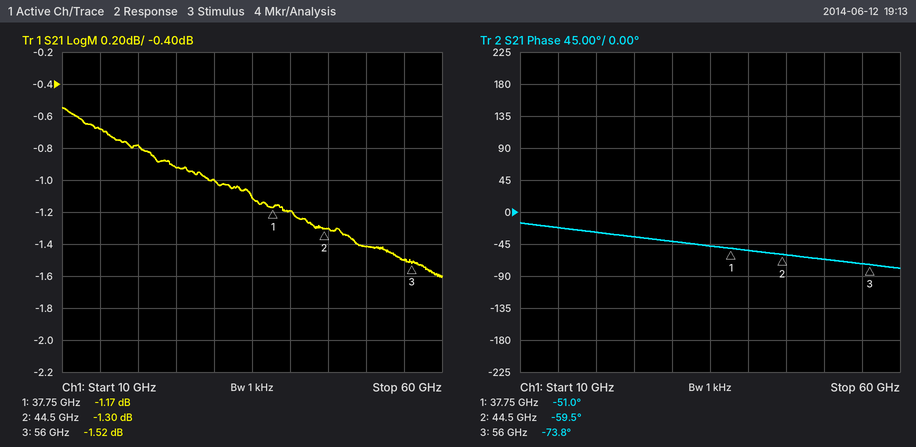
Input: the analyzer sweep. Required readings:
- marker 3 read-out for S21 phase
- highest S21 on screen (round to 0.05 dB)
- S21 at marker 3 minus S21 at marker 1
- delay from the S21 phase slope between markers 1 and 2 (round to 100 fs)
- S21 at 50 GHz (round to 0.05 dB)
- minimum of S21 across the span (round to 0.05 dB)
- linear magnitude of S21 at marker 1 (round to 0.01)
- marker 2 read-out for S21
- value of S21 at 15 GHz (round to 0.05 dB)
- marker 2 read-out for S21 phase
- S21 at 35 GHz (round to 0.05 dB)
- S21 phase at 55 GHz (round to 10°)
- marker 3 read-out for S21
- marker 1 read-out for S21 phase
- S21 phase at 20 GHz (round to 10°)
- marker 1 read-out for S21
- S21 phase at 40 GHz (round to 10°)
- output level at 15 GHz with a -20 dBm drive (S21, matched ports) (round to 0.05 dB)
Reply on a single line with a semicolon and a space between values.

-73.8°; -0.55 dB; -0.35 dB; 3.5 ps; -1.40 dB; -1.60 dB; 0.87; -1.30 dB; -0.70 dB; -59.5°; -1.10 dB; -70°; -1.52 dB; -51.0°; -30°; -1.17 dB; -50°; -20.70 dBm
